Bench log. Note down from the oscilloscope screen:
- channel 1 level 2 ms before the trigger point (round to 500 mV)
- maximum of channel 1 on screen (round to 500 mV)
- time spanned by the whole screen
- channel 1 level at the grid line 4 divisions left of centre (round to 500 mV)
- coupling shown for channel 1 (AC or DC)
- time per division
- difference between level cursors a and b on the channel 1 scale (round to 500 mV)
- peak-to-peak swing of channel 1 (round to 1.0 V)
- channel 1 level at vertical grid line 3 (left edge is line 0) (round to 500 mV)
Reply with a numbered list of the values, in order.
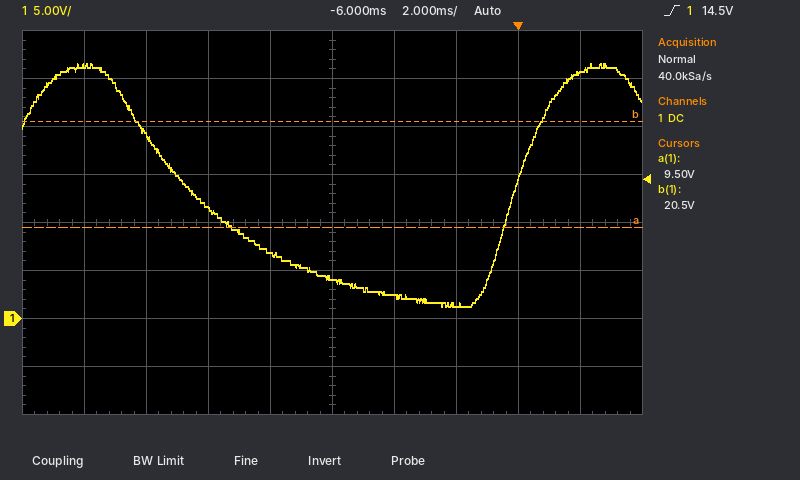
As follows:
1. 1.5 V
2. 26.5 V
3. 20 ms
4. 26.5 V
5. DC
6. 2 ms
7. 11.0 V
8. 25.0 V
9. 11.5 V
